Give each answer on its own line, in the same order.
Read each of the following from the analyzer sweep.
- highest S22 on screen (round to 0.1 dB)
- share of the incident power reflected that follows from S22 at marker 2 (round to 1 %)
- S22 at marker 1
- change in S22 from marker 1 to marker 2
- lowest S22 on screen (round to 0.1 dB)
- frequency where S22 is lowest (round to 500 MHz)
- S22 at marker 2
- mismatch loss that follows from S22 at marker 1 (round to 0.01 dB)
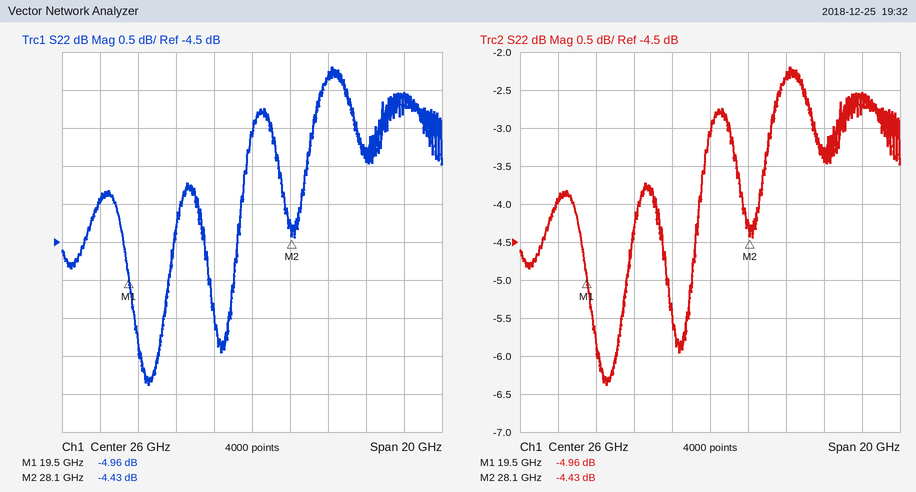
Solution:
-2.2 dB
36 %
-4.96 dB
0.53 dB
-6.4 dB
20.5 GHz
-4.43 dB
1.67 dB
